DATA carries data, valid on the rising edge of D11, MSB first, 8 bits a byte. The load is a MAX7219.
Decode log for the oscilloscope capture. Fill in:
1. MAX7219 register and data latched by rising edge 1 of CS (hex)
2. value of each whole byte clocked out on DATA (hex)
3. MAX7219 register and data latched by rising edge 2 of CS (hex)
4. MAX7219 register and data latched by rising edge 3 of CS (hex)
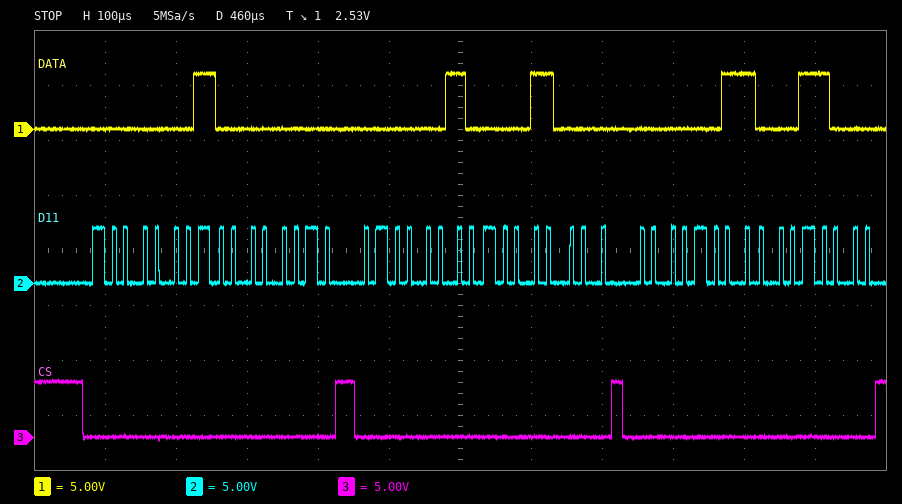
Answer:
register 0x1, data 0x00
0x01 0x00 0x02 0x18 0x03 0x18
register 0x2, data 0x18
register 0x3, data 0x18
